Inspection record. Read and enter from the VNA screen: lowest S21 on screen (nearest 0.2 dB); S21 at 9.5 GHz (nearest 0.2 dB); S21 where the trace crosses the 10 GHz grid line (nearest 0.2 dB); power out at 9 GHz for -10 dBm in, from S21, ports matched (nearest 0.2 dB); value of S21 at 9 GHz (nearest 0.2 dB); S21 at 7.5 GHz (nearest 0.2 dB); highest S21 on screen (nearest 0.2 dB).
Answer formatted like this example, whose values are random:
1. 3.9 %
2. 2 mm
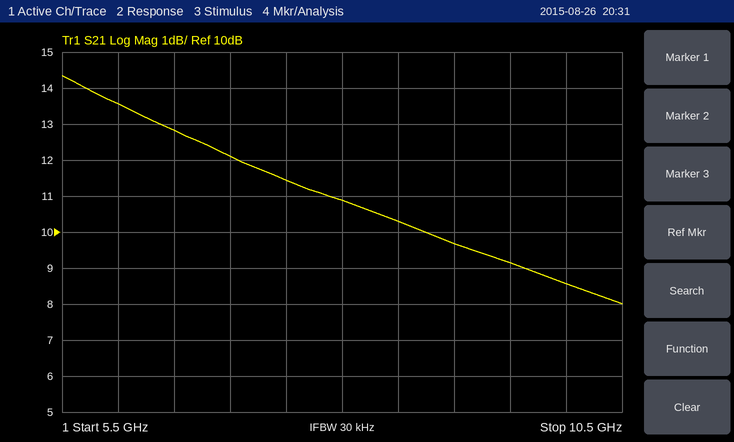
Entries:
1. 8.0 dB
2. 9.2 dB
3. 8.6 dB
4. -0.4 dBm
5. 9.6 dB
6. 11.4 dB
7. 14.4 dB
